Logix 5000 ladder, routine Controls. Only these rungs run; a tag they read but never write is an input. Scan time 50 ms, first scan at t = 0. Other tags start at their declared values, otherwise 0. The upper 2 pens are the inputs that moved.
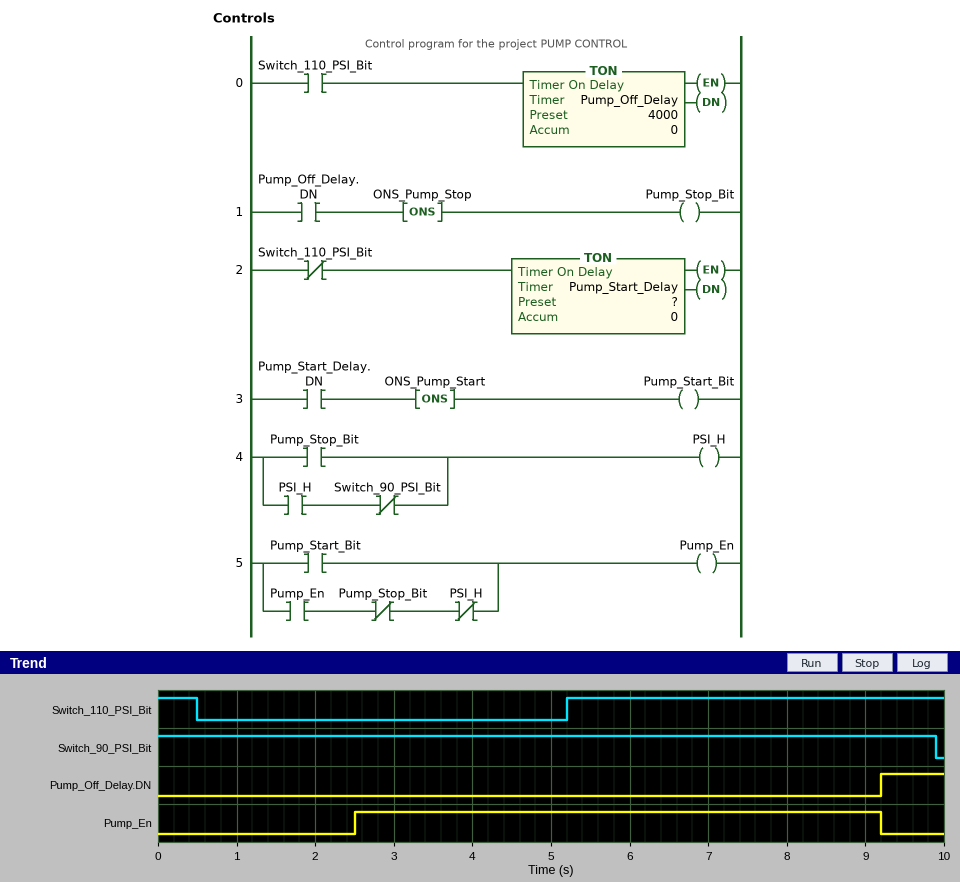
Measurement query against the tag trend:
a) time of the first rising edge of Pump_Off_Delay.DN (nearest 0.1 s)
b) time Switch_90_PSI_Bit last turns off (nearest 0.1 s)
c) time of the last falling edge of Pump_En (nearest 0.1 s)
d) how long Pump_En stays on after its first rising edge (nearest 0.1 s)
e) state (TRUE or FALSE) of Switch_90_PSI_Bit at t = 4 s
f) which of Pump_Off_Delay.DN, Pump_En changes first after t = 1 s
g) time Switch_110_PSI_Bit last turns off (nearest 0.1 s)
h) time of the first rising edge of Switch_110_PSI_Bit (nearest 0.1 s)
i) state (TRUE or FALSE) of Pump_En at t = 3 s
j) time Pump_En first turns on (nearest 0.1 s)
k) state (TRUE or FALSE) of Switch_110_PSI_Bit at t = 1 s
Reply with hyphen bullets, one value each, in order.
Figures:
- 9.2 s
- 9.9 s
- 9.2 s
- 6.7 s
- TRUE
- Pump_En
- 0.5 s
- 5.2 s
- TRUE
- 2.5 s
- FALSE
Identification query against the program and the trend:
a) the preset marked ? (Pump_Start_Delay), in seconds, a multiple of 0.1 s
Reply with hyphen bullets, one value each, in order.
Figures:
- 2.0 s
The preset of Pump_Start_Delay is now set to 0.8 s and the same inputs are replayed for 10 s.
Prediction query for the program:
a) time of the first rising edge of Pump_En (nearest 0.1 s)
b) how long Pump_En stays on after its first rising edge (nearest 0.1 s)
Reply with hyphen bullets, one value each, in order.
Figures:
- 1.3 s
- 7.9 s
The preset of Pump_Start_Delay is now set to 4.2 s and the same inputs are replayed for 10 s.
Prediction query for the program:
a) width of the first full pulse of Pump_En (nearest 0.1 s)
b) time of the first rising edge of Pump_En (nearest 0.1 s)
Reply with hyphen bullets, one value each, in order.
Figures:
- 4.5 s
- 4.7 s
